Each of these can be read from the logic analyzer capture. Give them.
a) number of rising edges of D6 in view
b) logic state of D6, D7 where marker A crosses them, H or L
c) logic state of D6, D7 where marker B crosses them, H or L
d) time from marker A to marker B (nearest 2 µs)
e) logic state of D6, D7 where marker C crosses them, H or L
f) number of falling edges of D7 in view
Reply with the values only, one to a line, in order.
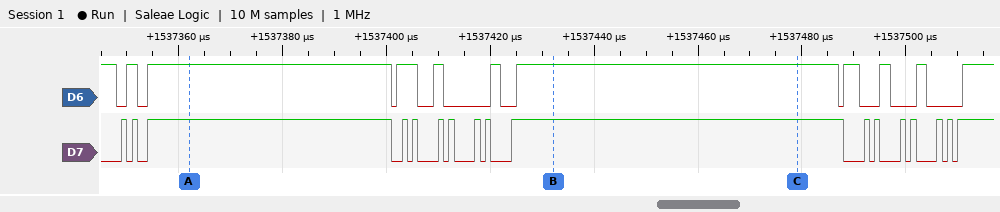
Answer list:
10
D6=H, D7=H
D6=H, D7=H
70 µs
D6=H, D7=H
16
